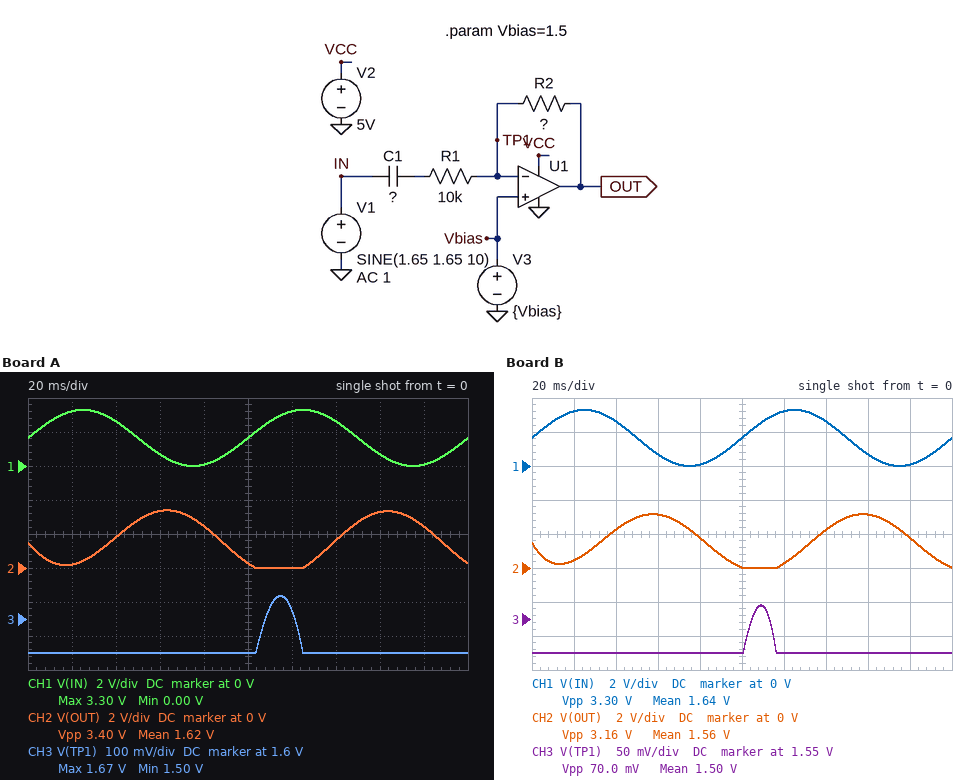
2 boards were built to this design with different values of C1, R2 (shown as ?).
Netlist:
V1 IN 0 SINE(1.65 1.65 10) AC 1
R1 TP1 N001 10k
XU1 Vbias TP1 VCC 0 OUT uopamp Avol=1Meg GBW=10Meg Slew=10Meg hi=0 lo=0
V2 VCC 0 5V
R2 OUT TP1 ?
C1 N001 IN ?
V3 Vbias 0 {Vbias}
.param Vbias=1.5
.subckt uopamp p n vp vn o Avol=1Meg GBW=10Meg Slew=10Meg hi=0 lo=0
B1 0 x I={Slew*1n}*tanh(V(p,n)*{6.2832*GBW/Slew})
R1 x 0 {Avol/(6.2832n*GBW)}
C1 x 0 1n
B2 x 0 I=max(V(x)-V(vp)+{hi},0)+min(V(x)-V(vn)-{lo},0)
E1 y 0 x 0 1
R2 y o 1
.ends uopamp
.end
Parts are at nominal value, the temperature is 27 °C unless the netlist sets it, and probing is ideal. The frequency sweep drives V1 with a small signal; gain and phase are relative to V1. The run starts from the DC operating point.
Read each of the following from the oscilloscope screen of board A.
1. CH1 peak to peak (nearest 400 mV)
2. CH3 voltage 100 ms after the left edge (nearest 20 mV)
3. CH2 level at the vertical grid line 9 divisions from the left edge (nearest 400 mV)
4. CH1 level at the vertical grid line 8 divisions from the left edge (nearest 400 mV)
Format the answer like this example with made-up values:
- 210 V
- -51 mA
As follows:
- 3.2 V
- 1.50 V
- 2.4 V
- 800 mV
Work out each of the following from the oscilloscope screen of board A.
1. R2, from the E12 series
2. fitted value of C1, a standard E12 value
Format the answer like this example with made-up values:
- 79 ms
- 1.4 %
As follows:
- 15 kΩ
- 1.8 µF
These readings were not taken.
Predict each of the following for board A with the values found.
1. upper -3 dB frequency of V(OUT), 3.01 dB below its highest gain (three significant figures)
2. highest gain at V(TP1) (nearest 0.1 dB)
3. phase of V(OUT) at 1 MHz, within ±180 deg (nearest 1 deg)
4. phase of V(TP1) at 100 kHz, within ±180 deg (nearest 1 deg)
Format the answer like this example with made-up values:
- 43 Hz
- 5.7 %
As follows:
- 4.00 MHz
- -4.4 dB
- 166 deg
- 89 deg
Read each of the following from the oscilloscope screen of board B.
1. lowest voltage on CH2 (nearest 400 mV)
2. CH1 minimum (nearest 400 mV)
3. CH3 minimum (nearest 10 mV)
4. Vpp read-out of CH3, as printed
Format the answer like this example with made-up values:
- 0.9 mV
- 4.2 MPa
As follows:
- 0 V
- 0 V
- 1.50 V
- 70.0 mV
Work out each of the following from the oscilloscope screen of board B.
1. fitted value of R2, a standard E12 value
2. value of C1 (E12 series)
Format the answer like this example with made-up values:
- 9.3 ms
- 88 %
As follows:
- 22 kΩ
- 820 nF
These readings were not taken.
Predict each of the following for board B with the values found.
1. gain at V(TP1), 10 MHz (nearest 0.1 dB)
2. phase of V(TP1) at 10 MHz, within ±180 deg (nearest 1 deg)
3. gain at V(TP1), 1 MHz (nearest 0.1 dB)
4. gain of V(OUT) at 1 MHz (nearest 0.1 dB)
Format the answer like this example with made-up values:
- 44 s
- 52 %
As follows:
- -3.7 dB
- 17 deg
- -13.6 dB
- 6.4 dB
